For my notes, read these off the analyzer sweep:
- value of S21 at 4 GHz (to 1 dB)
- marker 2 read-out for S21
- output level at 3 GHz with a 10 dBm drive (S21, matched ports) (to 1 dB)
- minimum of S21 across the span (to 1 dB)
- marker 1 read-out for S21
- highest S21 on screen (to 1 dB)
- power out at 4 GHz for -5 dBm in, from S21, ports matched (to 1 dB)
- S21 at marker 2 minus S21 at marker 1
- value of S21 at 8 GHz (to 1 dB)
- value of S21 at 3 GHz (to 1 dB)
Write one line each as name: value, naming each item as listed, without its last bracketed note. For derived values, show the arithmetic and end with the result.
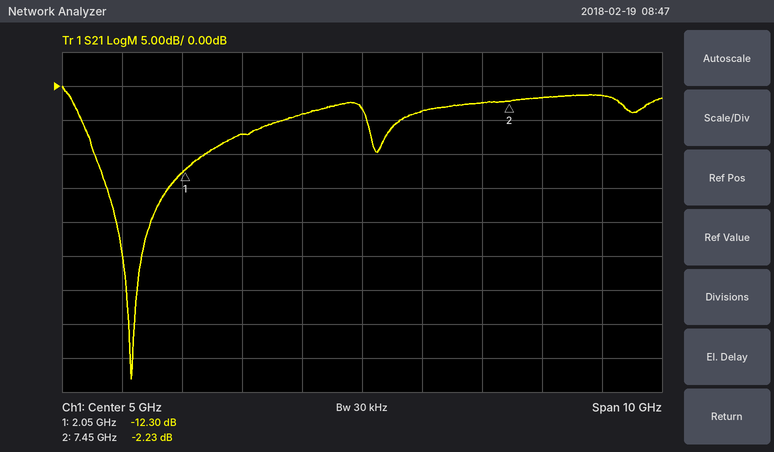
value of S21 at 4 GHz: -4 dB
marker 2 read-out for S21: -2.23 dB
output level at 3 GHz with a 10 dBm drive (S21, matched ports): 10 dBm + (-7 dB) = 3 dBm
minimum of S21 across the span: -43 dB
marker 1 read-out for S21: -12.30 dB
highest S21 on screen: 0 dB
power out at 4 GHz for -5 dBm in, from S21, ports matched: -5 dBm + (-4 dB) = -9 dBm
S21 at marker 2 minus S21 at marker 1: -2.23 − (-12.3) = 10.07 dB
value of S21 at 8 GHz: -2 dB
value of S21 at 3 GHz: -7 dB
